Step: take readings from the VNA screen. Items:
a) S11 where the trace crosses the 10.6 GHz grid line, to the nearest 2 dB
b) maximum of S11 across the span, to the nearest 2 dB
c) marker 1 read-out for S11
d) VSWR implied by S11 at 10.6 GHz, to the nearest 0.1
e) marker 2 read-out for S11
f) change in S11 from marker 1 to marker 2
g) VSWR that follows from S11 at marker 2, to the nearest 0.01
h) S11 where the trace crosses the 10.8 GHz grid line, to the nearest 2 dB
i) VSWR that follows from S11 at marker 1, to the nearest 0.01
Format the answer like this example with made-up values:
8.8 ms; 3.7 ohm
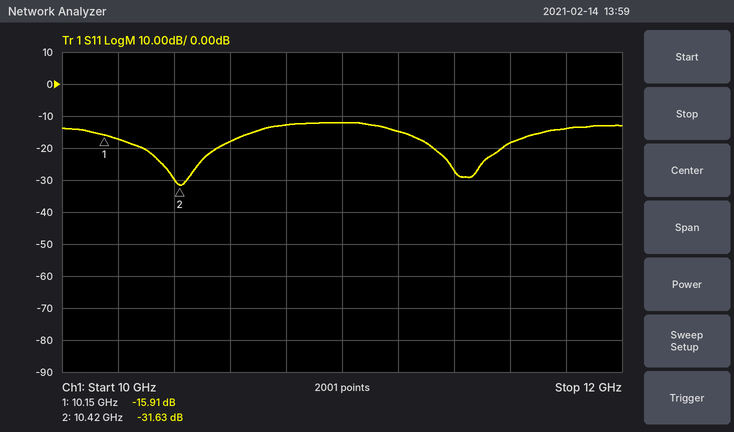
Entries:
-18 dB; -12 dB; -15.91 dB; 1.3; -31.63 dB; -15.72 dB; 1.05; -12 dB; 1.38
